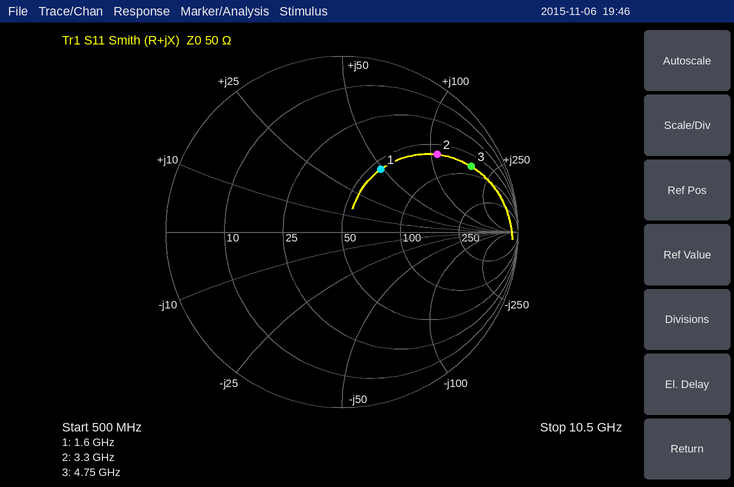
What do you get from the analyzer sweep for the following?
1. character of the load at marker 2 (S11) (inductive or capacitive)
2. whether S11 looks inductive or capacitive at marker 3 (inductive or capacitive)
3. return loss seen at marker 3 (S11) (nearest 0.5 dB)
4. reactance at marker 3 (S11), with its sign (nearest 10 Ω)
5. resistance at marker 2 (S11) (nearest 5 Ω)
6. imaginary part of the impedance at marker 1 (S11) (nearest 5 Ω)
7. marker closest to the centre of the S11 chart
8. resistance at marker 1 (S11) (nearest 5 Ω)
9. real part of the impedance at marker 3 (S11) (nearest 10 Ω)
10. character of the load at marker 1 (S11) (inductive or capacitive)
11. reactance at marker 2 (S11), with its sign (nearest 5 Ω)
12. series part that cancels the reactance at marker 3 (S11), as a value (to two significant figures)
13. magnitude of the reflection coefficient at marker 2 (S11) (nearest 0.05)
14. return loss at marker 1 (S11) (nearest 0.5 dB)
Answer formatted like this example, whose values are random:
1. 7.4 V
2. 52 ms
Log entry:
1. inductive
2. inductive
3. 1.5 dB
4. +180 Ω
5. 65 Ω
6. +50 Ω
7. marker 1
8. 55 Ω
9. 80 Ω
10. inductive
11. +110 Ω
12. 190 fF
13. 0.70
14. 7.5 dB
